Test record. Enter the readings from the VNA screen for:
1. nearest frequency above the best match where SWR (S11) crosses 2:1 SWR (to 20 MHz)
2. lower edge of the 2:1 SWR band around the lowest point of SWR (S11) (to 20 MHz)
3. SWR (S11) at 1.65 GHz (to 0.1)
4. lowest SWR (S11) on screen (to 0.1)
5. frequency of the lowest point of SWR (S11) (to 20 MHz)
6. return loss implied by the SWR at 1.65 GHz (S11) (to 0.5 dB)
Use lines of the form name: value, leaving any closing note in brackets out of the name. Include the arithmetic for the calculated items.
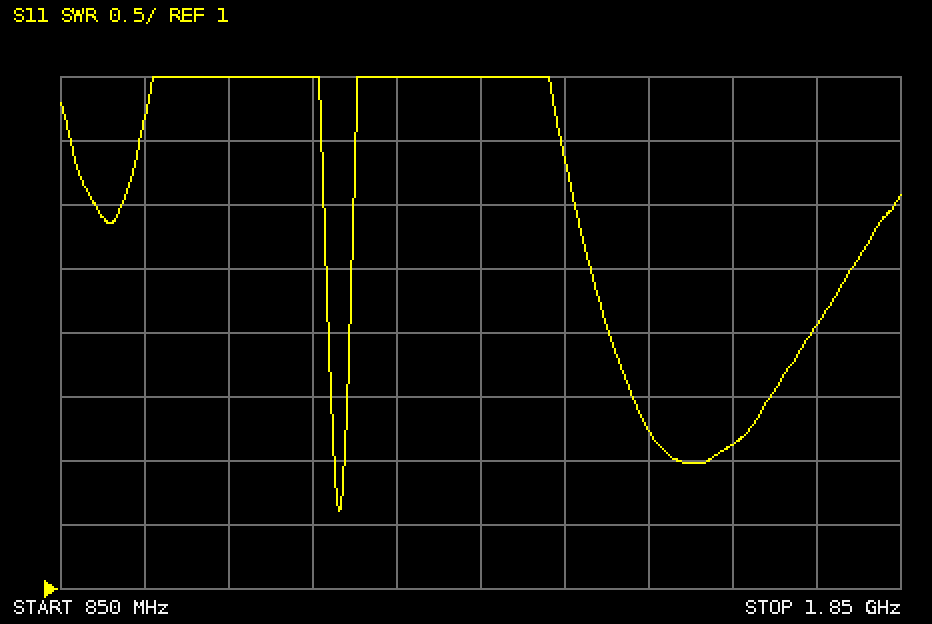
nearest frequency above the best match where SWR (S11) crosses 2:1 SWR: 1.18 GHz
lower edge of the 2:1 SWR band around the lowest point of SWR (S11): 1.18 GHz
SWR (S11) at 1.65 GHz: 2.1
lowest SWR (S11) on screen: 1.6
frequency of the lowest point of SWR (S11): 1.18 GHz
return loss implied by the SWR at 1.65 GHz (S11): −20 log10((2.1 − 1)/(2.1 + 1)) ≈ 9.0 dB
